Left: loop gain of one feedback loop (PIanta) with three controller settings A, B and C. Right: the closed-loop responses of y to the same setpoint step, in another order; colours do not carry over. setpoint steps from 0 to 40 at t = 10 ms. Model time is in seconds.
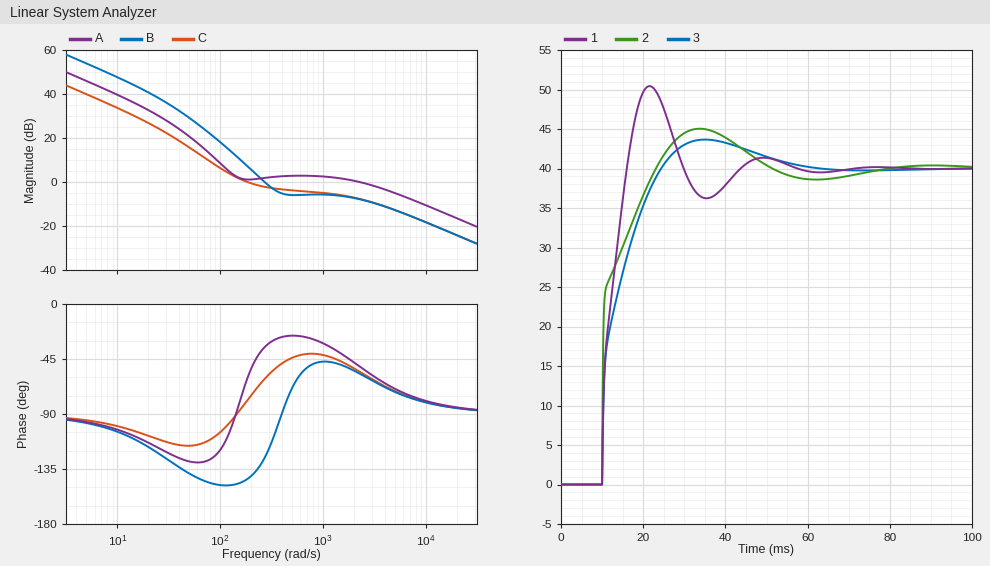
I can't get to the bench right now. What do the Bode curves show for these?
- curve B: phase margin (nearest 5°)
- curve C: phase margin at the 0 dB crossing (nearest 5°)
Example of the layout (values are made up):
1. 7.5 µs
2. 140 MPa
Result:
1. 55°
2. 100°
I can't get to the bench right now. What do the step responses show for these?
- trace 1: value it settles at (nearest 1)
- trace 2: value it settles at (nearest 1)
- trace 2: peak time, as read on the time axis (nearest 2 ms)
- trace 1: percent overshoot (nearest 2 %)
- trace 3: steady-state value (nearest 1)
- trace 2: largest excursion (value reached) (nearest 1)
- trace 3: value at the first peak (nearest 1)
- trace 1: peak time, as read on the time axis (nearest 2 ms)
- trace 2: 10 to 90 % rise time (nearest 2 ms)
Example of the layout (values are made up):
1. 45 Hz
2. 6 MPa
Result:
1. 40
2. 40
3. 34 ms
4. 26 %
5. 40
6. 45
7. 44
8. 22 ms
9. 10 ms
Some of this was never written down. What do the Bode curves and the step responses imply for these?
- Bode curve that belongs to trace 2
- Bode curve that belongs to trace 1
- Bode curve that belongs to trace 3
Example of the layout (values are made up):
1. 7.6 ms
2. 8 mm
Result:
1. A
2. B
3. C
